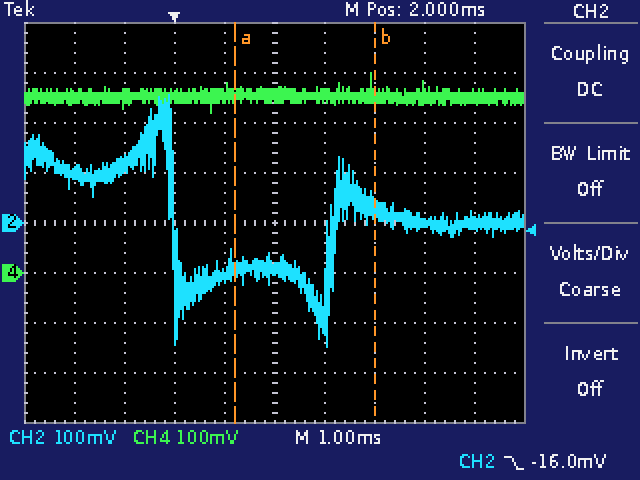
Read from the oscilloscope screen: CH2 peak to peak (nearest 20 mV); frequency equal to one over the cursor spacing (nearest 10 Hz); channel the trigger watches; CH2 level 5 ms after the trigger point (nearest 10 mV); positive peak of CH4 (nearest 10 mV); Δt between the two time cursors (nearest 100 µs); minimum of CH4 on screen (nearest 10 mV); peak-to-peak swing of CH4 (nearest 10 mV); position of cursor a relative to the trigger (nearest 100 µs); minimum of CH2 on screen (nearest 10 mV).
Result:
500 mV
360 Hz
CH2
0 mV
400 mV
2.8 ms
320 mV
80 mV
+1.2 ms
-250 mV
